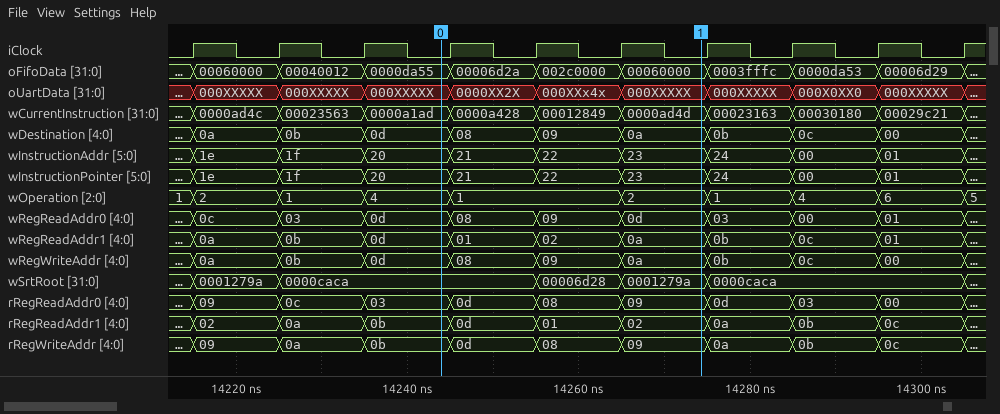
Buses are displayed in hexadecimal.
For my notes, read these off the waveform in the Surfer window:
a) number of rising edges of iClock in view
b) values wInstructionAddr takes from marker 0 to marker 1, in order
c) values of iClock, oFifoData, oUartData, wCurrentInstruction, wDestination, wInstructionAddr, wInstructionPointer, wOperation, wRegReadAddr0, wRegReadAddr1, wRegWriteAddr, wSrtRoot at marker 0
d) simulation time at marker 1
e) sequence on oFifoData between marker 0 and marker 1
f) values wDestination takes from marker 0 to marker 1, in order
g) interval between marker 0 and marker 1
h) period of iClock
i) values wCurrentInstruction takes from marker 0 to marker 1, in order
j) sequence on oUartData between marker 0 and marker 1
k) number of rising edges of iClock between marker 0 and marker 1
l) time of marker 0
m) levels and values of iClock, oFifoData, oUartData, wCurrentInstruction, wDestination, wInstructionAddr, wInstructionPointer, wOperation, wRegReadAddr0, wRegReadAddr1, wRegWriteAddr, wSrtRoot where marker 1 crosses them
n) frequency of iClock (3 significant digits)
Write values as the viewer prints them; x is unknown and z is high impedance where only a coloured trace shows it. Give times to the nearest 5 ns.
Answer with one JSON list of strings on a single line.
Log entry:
["10", "20, 21, 22, 23", "iClock=0, oFifoData=0000da55, oUartData=000XXXXX, wCurrentInstruction=0000a1ad, wDestination=0d, wInstructionAddr=20, wInstructionPointer=20, wOperation=4, wRegReadAddr0=0d, wRegReadAddr1=0d, wRegWriteAddr=0d, wSrtRoot=0000caca", "14275 ns", "0000da55, 00006d2a, 002c0000, 00060000", "0d, 08, 09, 0a", "30 ns", "10 ns", "0000a1ad, 0000a428, 00012849, 0000ad4d", "000XXXXX, 0000XX2X, 000XXx4x, 000XXXXX", "3", "14245 ns", "iClock=0, oFifoData=00060000, oUartData=000XXXXX, wCurrentInstruction=0000ad4d, wDestination=0a, wInstructionAddr=23, wInstructionPointer=23, wOperation=2, wRegReadAddr0=0d, wRegReadAddr1=0a, wRegWriteAddr=0a, wSrtRoot=0001279a", "100 MHz"]
